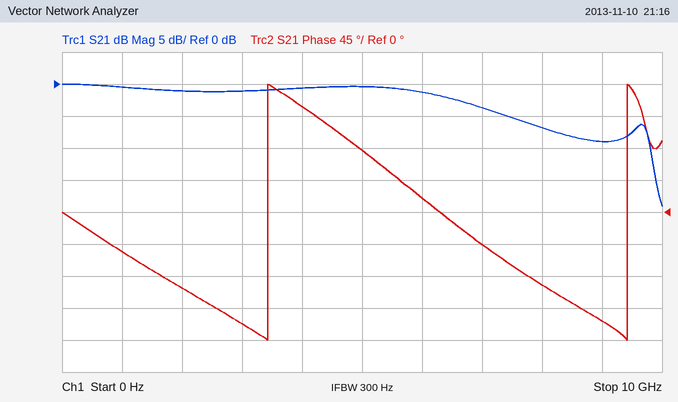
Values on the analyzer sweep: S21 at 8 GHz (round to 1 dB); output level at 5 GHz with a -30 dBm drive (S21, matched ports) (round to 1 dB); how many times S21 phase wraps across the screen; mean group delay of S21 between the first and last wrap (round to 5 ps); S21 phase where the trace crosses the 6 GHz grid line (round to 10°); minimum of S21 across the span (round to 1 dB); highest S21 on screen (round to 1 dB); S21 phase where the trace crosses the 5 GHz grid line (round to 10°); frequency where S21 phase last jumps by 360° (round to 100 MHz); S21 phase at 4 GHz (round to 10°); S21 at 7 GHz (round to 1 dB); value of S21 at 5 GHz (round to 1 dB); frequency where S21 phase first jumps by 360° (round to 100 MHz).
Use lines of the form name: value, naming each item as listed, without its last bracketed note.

S21 at 8 GHz: -7 dB
output level at 5 GHz with a -30 dBm drive (S21, matched ports): -30 dBm
how many times S21 phase wraps across the screen: 2
mean group delay of S21 between the first and last wrap: 165 ps
S21 phase where the trace crosses the 6 GHz grid line: 20°
minimum of S21 across the span: -19 dB
highest S21 on screen: 0 dB
S21 phase where the trace crosses the 5 GHz grid line: 90°
frequency where S21 phase last jumps by 360°: 9.4 GHz
S21 phase at 4 GHz: 150°
S21 at 7 GHz: -4 dB
value of S21 at 5 GHz: 0 dB
frequency where S21 phase first jumps by 360°: 3.4 GHz
